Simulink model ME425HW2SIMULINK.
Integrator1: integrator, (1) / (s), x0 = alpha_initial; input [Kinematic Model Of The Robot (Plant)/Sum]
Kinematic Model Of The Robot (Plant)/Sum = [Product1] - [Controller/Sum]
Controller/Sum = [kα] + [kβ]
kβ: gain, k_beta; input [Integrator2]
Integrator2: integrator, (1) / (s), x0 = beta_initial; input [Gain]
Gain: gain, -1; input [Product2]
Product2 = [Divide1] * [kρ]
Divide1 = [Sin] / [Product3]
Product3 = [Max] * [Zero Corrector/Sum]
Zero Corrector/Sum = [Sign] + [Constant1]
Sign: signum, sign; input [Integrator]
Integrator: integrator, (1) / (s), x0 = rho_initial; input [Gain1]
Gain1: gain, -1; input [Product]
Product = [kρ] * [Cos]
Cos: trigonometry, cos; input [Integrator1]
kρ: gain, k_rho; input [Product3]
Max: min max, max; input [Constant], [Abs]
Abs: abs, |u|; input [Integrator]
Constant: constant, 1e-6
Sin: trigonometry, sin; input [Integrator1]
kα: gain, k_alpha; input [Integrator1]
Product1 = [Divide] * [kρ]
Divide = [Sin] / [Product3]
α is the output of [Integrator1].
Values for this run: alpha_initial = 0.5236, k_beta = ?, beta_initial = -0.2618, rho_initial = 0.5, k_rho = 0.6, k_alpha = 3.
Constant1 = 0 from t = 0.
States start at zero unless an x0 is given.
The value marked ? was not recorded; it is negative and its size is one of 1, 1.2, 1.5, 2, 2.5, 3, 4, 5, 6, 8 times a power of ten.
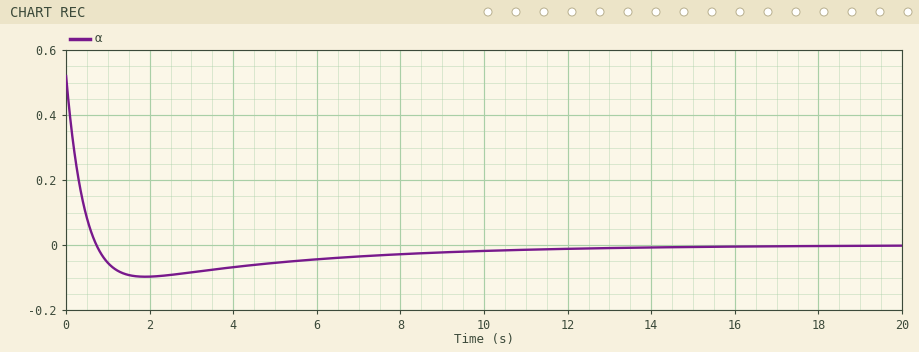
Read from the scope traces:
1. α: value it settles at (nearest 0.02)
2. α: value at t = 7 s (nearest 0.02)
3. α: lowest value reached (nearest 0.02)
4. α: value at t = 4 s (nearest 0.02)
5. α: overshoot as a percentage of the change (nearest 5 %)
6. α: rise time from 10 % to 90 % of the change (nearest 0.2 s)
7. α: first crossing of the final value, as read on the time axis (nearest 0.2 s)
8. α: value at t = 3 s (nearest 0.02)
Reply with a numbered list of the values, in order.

1. 0.00
2. -0.04
3. -0.10
4. -0.06
5. 20 %
6. 0.6 s
7. 0.8 s
8. -0.08
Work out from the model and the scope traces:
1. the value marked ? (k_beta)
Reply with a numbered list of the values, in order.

1. -0.8
